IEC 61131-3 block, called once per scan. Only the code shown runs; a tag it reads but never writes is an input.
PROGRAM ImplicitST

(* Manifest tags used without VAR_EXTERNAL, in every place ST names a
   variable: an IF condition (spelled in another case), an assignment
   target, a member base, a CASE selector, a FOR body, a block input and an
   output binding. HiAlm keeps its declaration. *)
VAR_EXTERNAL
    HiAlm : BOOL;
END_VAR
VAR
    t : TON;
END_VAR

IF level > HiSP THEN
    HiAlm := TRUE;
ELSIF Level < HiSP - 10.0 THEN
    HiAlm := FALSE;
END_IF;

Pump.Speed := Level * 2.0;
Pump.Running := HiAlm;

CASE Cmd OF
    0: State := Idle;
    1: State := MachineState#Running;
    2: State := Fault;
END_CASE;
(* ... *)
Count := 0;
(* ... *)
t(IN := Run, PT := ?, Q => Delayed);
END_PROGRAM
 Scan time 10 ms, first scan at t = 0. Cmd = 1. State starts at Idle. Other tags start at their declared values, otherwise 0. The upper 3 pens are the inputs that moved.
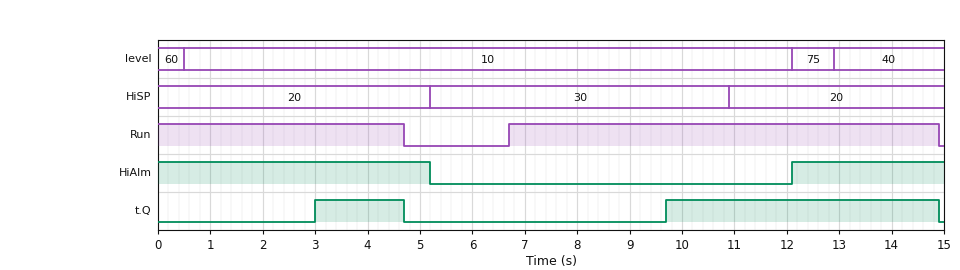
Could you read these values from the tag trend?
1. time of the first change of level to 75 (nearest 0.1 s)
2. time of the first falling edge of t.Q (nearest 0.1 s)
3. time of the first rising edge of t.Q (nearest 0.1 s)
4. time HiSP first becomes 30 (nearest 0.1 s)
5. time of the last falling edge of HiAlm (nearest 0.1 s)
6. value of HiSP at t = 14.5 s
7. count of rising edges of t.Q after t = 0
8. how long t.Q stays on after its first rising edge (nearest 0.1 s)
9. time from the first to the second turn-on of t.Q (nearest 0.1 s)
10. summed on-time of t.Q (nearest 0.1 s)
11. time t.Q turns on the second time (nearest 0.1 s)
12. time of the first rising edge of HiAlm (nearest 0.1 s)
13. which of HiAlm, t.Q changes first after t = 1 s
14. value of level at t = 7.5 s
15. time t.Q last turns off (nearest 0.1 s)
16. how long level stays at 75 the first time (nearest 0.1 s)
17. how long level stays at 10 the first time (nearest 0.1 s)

12.1 s
4.7 s
3.0 s
5.2 s
5.2 s
20
2
1.7 s
6.7 s
6.9 s
9.7 s
12.1 s
t.Q
10
14.9 s
0.8 s
11.6 s
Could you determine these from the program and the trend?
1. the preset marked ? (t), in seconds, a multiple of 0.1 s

3.0 s
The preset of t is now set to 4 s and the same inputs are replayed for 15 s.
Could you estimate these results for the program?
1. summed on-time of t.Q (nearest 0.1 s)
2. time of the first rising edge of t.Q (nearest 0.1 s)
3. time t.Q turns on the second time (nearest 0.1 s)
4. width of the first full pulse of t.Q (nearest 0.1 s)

4.9 s
4.0 s
10.7 s
0.7 s
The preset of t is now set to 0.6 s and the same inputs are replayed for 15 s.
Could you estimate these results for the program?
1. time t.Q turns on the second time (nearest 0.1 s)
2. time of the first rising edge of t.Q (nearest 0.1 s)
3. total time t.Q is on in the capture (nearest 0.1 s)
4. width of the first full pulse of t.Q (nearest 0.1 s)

7.3 s
0.6 s
11.7 s
4.1 s
